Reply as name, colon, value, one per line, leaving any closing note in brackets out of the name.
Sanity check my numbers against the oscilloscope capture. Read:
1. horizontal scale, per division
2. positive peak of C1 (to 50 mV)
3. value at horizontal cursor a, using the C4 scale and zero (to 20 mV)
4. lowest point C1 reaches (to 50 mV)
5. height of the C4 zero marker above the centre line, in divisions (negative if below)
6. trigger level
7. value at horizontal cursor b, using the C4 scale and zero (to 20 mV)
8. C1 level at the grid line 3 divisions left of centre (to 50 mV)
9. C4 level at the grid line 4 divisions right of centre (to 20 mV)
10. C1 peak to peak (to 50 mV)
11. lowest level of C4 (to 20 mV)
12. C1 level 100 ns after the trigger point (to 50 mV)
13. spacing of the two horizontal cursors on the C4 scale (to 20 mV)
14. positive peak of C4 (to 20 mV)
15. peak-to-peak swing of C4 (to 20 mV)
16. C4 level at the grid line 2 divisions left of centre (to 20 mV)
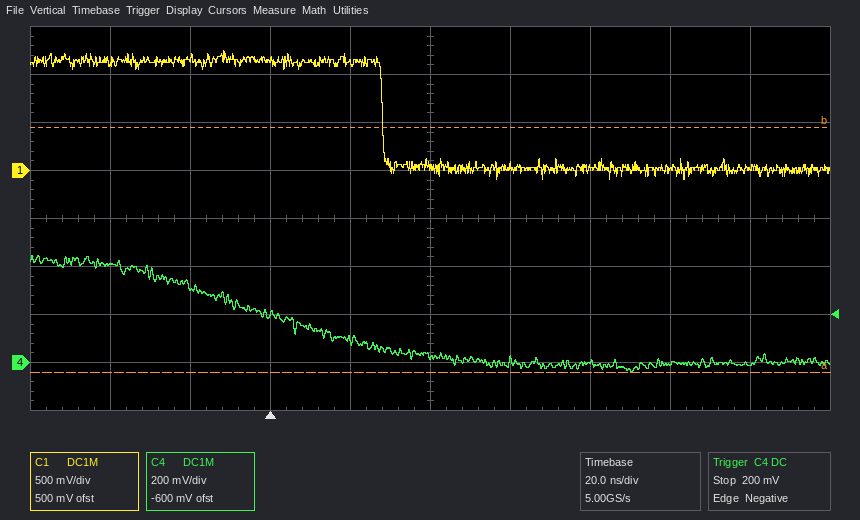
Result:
horizontal scale, per division: 20 ns
positive peak of C1: 1.25 V
value at horizontal cursor a, using the C4 scale and zero: -40 mV
lowest point C1 reaches: -100 mV
height of the C4 zero marker above the centre line, in divisions: -3.0 div
trigger level: 200 mV
value at horizontal cursor b, using the C4 scale and zero: 980 mV
C1 level at the grid line 3 divisions left of centre: 1.15 V
C4 level at the grid line 4 divisions right of centre: 0 mV
C1 peak to peak: 1.35 V
lowest level of C4: -40 mV
C1 level 100 ns after the trigger point: 0 mV
spacing of the two horizontal cursors on the C4 scale: 1.02 V
positive peak of C4: 440 mV
peak-to-peak swing of C4: 480 mV
C4 level at the grid line 2 divisions left of centre: 200 mV
